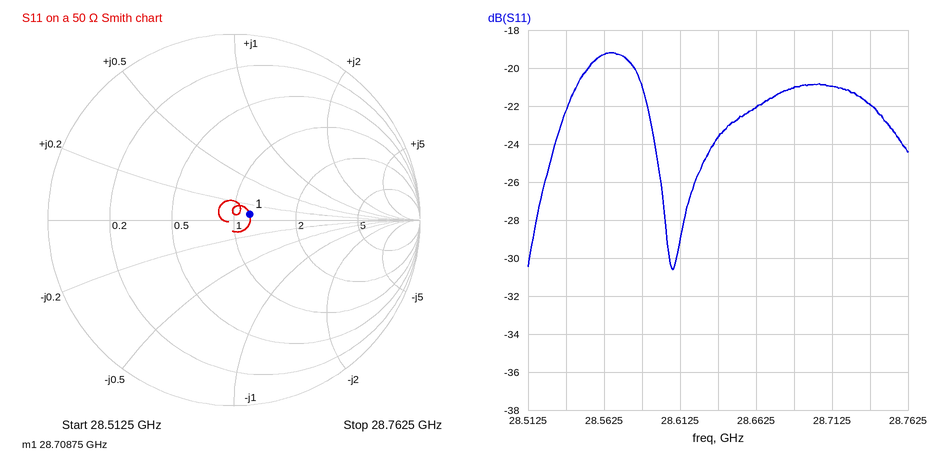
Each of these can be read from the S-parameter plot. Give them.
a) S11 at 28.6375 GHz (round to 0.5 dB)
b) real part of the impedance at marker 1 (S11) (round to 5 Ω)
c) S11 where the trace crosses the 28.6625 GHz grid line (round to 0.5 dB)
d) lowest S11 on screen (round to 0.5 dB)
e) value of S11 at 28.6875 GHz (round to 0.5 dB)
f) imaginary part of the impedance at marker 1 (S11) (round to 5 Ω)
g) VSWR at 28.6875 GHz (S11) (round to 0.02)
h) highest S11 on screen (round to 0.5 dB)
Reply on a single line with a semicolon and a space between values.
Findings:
-23.5 dB; 60 Ω; -22.0 dB; -30.5 dB; -21.0 dB; +5 Ω; 1.20; -19.0 dB
